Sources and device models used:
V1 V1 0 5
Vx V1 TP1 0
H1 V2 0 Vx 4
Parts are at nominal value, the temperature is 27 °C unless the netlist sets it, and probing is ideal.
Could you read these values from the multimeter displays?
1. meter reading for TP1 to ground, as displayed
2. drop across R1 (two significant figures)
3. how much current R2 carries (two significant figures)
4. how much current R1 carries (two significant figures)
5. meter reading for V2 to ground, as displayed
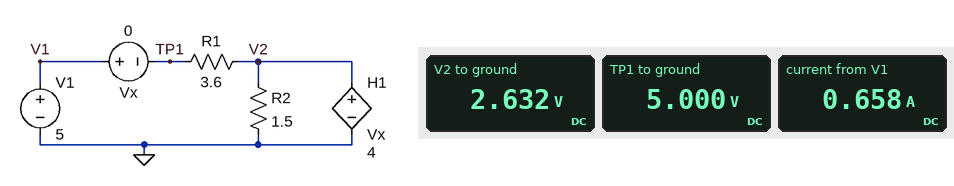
5.000 V
2.4 V
1.8 A
660 mA
2.632 V
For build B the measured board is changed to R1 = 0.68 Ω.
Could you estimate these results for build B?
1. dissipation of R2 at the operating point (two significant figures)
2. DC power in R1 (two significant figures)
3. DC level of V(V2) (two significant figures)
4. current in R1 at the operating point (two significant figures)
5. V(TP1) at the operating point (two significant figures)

12 W
780 mW
4.3 V
1.1 A
5.0 V
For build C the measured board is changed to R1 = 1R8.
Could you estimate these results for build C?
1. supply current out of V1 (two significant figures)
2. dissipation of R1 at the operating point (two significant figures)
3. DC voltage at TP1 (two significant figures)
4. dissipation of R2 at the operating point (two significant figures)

860 mA
1.3 W
5.0 V
7.9 W
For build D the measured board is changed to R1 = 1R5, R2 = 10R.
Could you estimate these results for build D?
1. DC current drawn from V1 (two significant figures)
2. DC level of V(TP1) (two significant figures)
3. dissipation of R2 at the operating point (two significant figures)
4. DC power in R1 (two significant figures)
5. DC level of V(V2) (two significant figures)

910 mA
5.0 V
1.3 W
1.2 W
3.6 V
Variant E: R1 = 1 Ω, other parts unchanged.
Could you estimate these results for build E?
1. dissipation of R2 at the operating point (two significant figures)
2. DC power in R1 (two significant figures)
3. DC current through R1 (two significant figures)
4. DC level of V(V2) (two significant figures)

11 W
1.0 W
1.0 A
4.0 V
